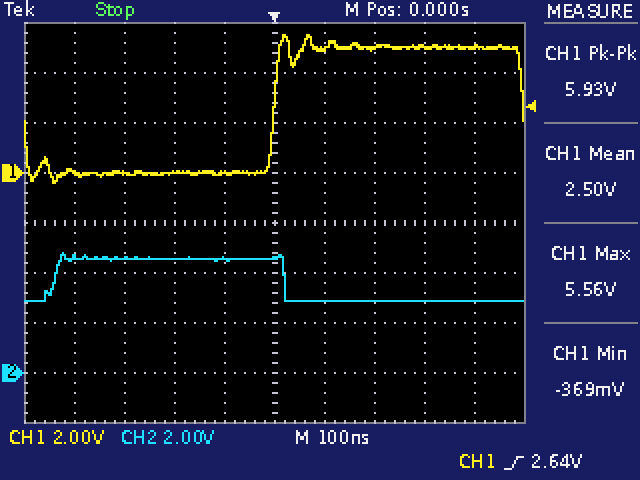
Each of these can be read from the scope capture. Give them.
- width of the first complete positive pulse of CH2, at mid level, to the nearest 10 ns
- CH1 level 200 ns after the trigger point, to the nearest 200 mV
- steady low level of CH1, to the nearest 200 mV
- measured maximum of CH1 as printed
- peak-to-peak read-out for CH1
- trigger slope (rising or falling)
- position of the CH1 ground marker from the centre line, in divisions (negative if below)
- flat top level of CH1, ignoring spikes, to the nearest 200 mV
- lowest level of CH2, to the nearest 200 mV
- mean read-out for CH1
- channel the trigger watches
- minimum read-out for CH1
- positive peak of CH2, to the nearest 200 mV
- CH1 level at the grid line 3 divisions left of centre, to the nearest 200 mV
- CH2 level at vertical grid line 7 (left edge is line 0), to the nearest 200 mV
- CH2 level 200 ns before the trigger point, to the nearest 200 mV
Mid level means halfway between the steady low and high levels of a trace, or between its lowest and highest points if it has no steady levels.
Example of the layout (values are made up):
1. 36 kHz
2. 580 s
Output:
1. 460 ns
2. 5.0 V
3. 0.0 V
4. 5.56 V
5. 5.93 V
6. rising
7. +1.0 div
8. 5.0 V
9. 2.8 V
10. 2.50 V
11. CH1
12. -369 mV
13. 4.8 V
14. 0.0 V
15. 2.8 V
16. 4.6 V
